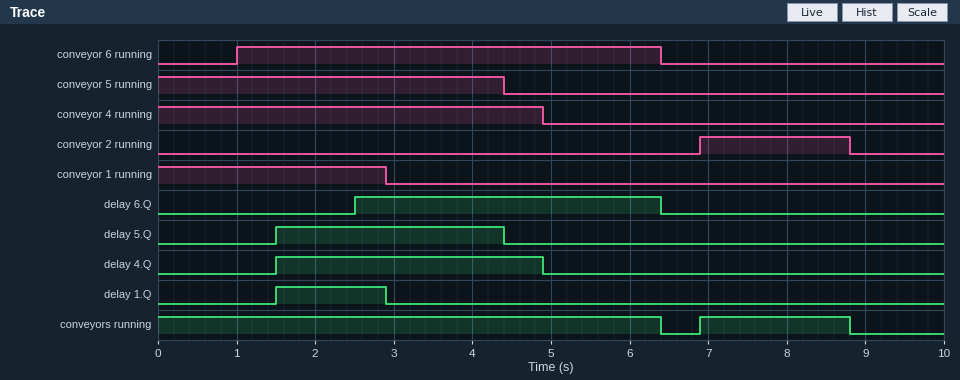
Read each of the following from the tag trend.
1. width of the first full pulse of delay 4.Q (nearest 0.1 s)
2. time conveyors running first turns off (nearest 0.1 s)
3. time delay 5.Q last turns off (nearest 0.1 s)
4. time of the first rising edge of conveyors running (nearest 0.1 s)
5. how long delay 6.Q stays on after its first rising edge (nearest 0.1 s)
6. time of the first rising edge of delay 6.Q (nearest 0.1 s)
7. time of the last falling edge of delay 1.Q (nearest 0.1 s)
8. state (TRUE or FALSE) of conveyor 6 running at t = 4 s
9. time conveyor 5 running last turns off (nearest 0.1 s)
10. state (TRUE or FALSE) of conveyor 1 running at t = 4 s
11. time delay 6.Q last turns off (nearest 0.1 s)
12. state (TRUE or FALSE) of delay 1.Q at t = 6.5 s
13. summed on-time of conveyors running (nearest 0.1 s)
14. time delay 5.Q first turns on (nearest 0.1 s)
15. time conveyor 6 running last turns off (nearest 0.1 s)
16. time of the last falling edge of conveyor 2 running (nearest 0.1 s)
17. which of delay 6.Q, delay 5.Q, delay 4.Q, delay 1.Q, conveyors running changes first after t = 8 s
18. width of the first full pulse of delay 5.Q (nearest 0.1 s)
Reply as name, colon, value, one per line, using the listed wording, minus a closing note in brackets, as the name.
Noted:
width of the first full pulse of delay 4.Q: 3.4 s
time conveyors running first turns off: 6.4 s
time delay 5.Q last turns off: 4.4 s
time of the first rising edge of conveyors running: 6.9 s
how long delay 6.Q stays on after its first rising edge: 3.9 s
time of the first rising edge of delay 6.Q: 2.5 s
time of the last falling edge of delay 1.Q: 2.9 s
state (TRUE or FALSE) of conveyor 6 running at t = 4 s: TRUE
time conveyor 5 running last turns off: 4.4 s
state (TRUE or FALSE) of conveyor 1 running at t = 4 s: FALSE
time delay 6.Q last turns off: 6.4 s
state (TRUE or FALSE) of delay 1.Q at t = 6.5 s: FALSE
summed on-time of conveyors running: 8.3 s
time delay 5.Q first turns on: 1.5 s
time conveyor 6 running last turns off: 6.4 s
time of the last falling edge of conveyor 2 running: 8.8 s
which of delay 6.Q, delay 5.Q, delay 4.Q, delay 1.Q, conveyors running changes first after t = 8 s: conveyors running
width of the first full pulse of delay 5.Q: 2.9 s
